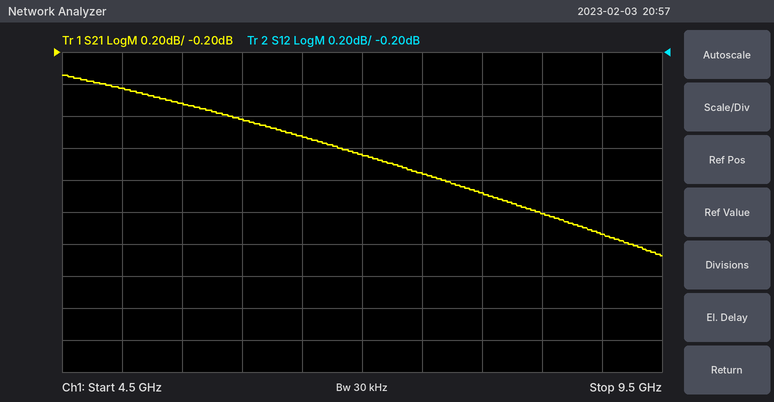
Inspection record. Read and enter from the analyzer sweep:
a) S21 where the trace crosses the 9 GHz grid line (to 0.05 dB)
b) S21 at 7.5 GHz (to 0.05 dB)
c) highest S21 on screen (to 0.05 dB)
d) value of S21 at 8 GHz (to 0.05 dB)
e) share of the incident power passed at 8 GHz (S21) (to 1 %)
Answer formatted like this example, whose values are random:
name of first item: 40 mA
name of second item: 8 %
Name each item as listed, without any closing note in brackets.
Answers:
S21 where the trace crosses the 9 GHz grid line: -1.35 dB
S21 at 7.5 GHz: -0.95 dB
highest S21 on screen: -0.35 dB
value of S21 at 8 GHz: -1.10 dB
share of the incident power passed at 8 GHz (S21): 78 %
